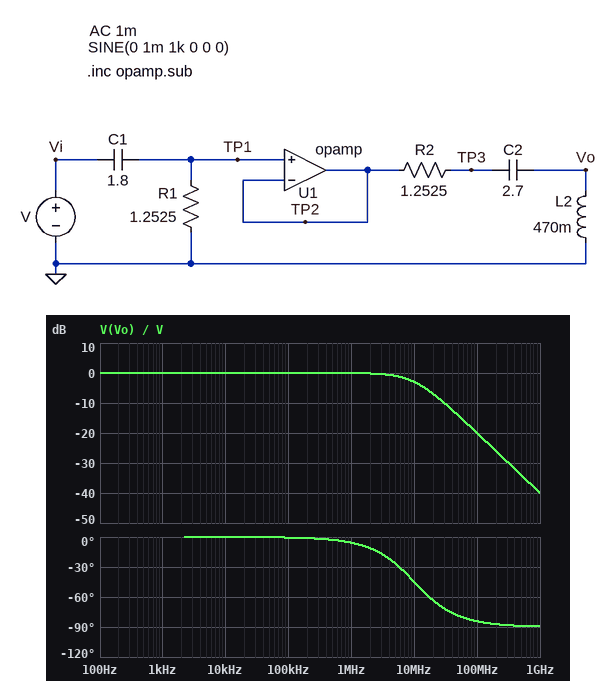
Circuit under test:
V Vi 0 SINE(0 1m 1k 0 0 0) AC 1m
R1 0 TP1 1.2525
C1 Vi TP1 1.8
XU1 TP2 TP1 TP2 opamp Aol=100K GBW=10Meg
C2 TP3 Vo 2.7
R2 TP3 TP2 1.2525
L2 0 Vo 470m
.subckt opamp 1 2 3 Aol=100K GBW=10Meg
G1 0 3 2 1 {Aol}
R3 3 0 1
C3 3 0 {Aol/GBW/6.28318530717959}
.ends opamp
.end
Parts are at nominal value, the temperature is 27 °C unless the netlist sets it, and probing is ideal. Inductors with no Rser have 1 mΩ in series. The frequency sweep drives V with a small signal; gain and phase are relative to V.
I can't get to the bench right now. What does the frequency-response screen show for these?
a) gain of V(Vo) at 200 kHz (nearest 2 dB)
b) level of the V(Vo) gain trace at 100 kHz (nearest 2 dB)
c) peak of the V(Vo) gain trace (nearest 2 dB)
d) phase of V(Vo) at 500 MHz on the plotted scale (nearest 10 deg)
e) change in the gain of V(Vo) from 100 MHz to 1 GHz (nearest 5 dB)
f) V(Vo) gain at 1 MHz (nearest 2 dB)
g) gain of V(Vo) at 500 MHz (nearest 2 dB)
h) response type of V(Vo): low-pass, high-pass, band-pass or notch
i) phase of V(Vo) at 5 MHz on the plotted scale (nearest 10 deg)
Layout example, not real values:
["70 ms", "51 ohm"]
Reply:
["0 dB", "0 dB", "0 dB", "-90 deg", "-20 dB", "0 dB", "-34 dB", "low-pass", "-30 deg"]
